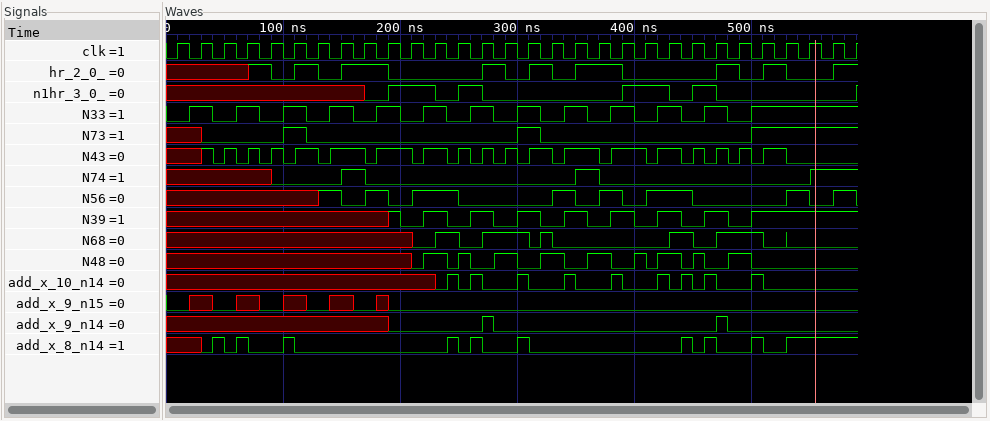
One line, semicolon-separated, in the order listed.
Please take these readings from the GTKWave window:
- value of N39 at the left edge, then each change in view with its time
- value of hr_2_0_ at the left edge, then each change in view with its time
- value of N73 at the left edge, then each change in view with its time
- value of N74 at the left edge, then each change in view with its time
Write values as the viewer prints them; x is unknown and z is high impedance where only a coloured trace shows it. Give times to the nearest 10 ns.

x, 1 at 190 ns, 0 at 200 ns, 1 at 220 ns, 0 at 240 ns, 1 at 260 ns, 0 at 280 ns, 1 at 300 ns, 0 at 320 ns, 1 at 340 ns, 0 at 360 ns, 1 at 380 ns, 0 at 400 ns, 1 at 420 ns, 0 at 440 ns, 1 at 460 ns, 0 at 480 ns, 1 at 500 ns; x, 1 at 70 ns, 0 at 90 ns, 1 at 110 ns, 0 at 130 ns, 1 at 150 ns, 0 at 190 ns, 1 at 270 ns, 0 at 290 ns, 1 at 310 ns, 0 at 330 ns, 1 at 350 ns, 0 at 390 ns, 1 at 470 ns, 0 at 490 ns, 1 at 510 ns, 0 at 530 ns, 1 at 570 ns; x, 0 at 30 ns, 1 at 100 ns, 0 at 120 ns, 1 at 300 ns, 0 at 320 ns, 1 at 500 ns; x, 0 at 90 ns, 1 at 150 ns, 0 at 170 ns, 1 at 350 ns, 0 at 370 ns, 1 at 550 ns
